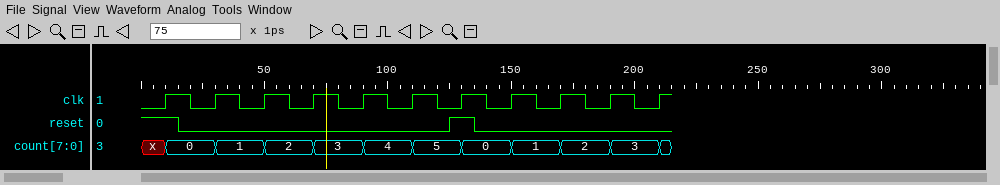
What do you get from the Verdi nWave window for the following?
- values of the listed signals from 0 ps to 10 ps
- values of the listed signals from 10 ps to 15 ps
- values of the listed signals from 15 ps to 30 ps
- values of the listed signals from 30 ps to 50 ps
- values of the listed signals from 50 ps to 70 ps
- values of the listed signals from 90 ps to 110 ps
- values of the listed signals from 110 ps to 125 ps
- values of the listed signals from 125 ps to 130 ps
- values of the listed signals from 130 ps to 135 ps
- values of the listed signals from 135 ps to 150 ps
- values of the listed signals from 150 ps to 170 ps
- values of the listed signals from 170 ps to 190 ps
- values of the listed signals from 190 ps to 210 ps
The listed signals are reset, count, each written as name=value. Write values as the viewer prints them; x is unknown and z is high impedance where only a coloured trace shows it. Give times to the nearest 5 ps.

reset=1, count=x
reset=1, count=0
reset=0, count=0
reset=0, count=1
reset=0, count=2
reset=0, count=4
reset=0, count=5
reset=1, count=5
reset=1, count=0
reset=0, count=0
reset=0, count=1
reset=0, count=2
reset=0, count=3
